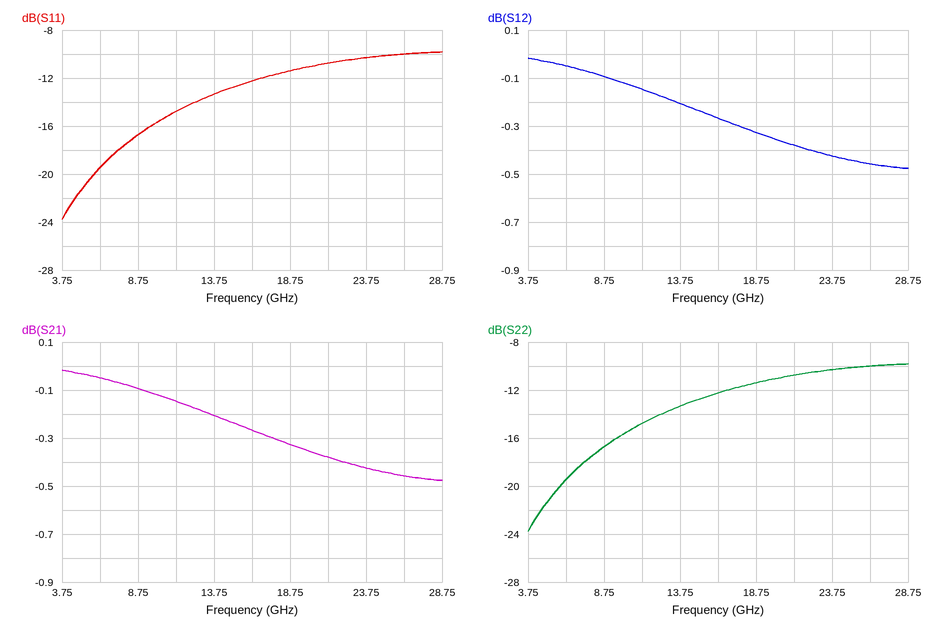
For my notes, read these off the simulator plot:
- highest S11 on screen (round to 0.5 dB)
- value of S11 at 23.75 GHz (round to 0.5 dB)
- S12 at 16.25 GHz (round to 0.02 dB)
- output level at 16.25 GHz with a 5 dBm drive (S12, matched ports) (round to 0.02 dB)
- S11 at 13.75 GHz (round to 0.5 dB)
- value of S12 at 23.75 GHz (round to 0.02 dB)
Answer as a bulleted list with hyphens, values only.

- -10.0 dB
- -10.5 dB
- -0.26 dB
- 4.74 dBm
- -13.5 dB
- -0.42 dB
